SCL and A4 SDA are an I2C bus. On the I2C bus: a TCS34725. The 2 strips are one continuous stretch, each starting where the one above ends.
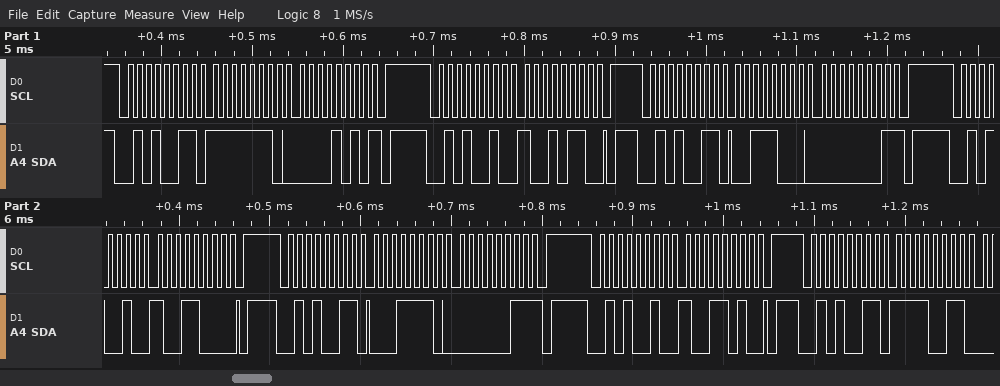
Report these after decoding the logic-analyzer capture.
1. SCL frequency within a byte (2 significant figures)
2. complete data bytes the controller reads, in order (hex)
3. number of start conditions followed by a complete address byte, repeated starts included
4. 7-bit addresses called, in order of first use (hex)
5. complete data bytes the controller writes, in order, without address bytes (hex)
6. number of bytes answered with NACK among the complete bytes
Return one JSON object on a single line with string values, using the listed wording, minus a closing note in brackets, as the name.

{"SCL frequency within a byte": "100 kHz", "complete data bytes the controller reads, in order": "FE 0A 38 01 1E 03 F3", "number of start conditions followed by a complete address byte, repeated starts included": "7", "7-bit addresses called, in order of first use": "0x29", "complete data bytes the controller writes, in order, without address bytes": "96 98 9A", "number of bytes answered with NACK among the complete bytes": "3"}
